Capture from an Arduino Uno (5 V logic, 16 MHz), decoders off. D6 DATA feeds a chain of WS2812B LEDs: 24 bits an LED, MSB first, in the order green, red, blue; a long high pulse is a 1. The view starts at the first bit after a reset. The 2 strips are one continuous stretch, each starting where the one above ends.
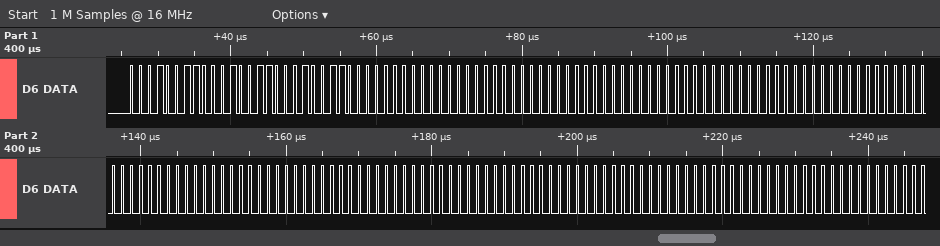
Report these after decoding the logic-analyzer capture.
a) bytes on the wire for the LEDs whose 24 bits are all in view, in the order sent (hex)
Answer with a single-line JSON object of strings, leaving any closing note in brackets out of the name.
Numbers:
{"bytes on the wire for the LEDs whose 24 bits are all in view, in the order sent": "13 13 13 00 00 00 00 00 00 00 00 00 00 00 00 00 00 00 00 00 00"}
